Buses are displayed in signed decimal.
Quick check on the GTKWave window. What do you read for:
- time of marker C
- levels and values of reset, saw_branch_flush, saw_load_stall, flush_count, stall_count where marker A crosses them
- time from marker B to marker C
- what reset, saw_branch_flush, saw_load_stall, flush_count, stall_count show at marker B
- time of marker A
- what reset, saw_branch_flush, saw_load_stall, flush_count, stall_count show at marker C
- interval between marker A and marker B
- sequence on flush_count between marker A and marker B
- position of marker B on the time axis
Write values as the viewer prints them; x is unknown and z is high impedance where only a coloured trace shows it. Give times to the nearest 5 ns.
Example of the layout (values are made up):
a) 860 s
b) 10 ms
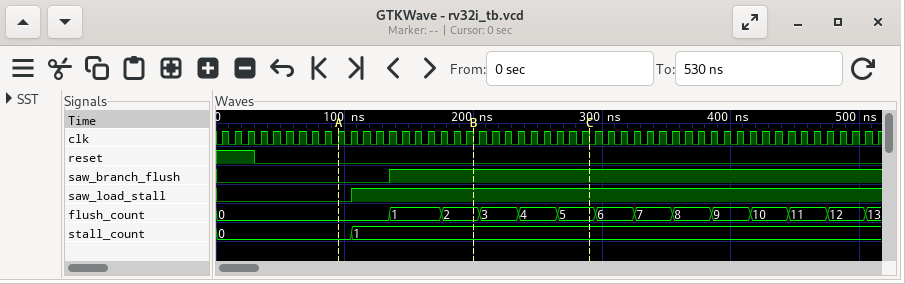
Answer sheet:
a) 290 ns
b) reset=0, saw_branch_flush=0, saw_load_stall=0, flush_count=0, stall_count=0
c) 90 ns
d) reset=0, saw_branch_flush=1, saw_load_stall=1, flush_count=2, stall_count=1
e) 95 ns
f) reset=0, saw_branch_flush=1, saw_load_stall=1, flush_count=5, stall_count=1
g) 105 ns
h) 0, 1, 2
i) 200 ns
